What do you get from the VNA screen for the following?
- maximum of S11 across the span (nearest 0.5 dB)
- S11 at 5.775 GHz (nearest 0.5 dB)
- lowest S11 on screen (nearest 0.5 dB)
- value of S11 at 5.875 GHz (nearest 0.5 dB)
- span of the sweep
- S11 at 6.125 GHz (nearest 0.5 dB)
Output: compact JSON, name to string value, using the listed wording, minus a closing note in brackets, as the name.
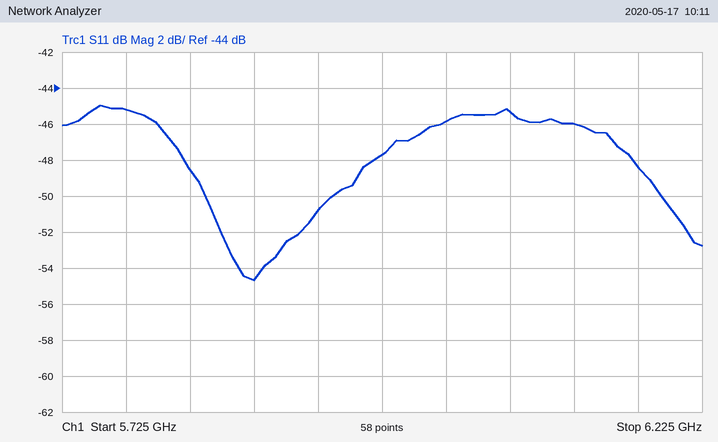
{"maximum of S11 across the span": "-45.0 dB", "S11 at 5.775 GHz": "-45.0 dB", "lowest S11 on screen": "-54.5 dB", "value of S11 at 5.875 GHz": "-54.5 dB", "span of the sweep": "500 MHz", "S11 at 6.125 GHz": "-46.0 dB"}
